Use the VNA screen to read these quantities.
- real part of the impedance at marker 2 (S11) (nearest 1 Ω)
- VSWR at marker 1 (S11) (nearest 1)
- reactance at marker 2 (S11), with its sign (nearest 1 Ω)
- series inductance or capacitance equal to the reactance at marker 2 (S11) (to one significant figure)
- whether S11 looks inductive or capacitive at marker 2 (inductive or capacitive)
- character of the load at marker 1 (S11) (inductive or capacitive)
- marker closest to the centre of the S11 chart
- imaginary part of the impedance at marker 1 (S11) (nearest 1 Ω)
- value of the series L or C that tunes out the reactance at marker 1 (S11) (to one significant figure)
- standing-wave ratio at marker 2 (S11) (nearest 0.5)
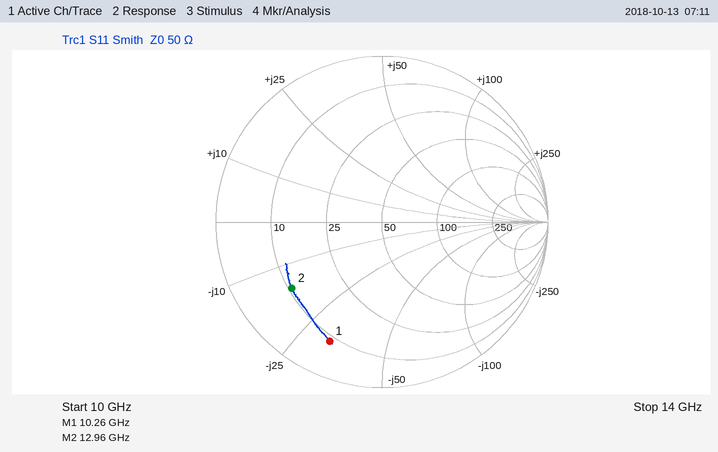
11 Ω
8
-16 Ω
800 fF
capacitive
capacitive
marker 2
-32 Ω
500 pH
5.0
